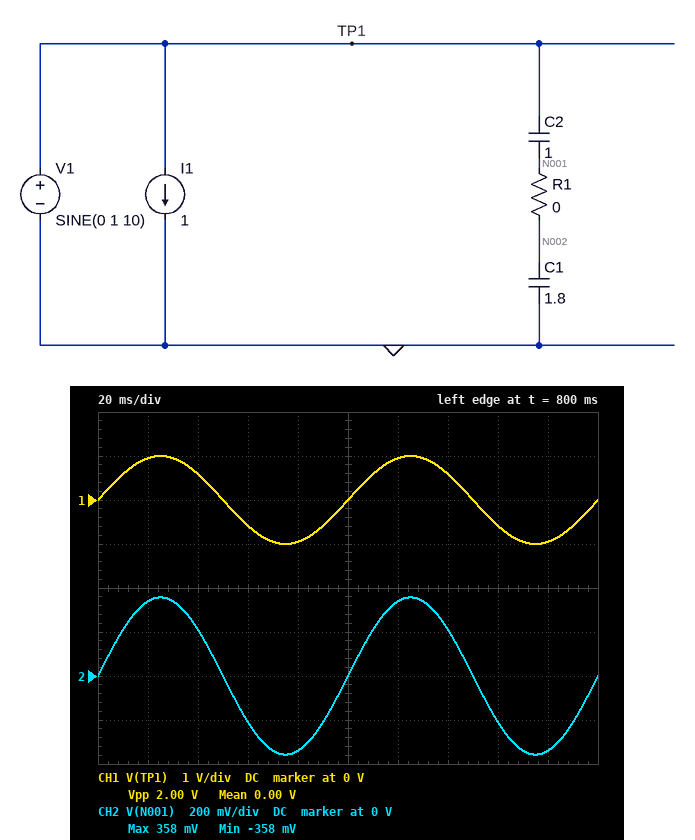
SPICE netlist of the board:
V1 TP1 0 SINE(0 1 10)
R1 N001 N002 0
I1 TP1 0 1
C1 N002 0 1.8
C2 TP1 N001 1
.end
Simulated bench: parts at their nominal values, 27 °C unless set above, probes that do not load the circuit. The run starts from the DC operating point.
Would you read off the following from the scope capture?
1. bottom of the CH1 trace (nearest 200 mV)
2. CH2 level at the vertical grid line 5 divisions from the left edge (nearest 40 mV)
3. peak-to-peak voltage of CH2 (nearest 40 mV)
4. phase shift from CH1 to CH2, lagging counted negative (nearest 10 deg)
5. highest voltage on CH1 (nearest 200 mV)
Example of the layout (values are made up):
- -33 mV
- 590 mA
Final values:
- -1.0 V
- 0 V
- 720 mV
- 0 deg
- 1.0 V
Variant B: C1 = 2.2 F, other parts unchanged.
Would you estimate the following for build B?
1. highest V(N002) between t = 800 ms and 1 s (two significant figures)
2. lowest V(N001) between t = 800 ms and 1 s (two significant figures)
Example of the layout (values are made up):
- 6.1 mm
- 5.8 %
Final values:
- 310 mV
- -310 mV
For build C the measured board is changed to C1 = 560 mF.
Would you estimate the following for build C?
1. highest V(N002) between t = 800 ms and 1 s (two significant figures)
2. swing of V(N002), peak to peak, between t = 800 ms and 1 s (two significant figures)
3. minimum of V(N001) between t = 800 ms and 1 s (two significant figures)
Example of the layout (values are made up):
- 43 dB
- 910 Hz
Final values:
- 640 mV
- 1.3 V
- -640 mV
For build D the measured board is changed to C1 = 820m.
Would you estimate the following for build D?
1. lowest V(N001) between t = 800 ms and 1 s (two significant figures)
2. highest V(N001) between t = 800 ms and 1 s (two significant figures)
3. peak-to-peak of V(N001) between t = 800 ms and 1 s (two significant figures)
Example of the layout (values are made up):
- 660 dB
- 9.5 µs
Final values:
- -550 mV
- 550 mV
- 1.1 V
